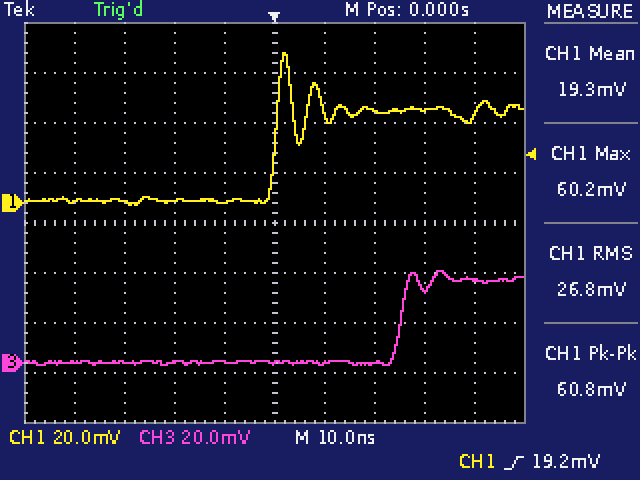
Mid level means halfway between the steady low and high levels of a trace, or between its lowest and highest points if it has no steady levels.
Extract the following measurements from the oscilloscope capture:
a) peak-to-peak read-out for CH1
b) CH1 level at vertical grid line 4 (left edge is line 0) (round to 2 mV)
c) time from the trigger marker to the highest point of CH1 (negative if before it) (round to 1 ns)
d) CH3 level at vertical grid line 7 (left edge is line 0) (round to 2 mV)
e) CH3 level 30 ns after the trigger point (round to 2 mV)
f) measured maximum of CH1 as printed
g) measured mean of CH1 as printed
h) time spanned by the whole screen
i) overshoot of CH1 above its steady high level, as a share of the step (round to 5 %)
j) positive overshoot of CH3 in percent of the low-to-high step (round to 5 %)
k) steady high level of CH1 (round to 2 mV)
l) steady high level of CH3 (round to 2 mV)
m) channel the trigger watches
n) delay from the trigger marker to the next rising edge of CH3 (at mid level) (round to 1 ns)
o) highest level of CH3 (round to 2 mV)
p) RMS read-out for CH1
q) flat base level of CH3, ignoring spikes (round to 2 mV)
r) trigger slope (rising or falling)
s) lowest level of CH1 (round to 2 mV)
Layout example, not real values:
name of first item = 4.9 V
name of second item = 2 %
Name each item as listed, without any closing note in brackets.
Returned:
peak-to-peak read-out for CH1 = 60.8 mV
CH1 level at vertical grid line 4 (left edge is line 0) = 0 mV
time from the trigger marker to the highest point of CH1 (negative if before it) = +2 ns
CH3 level at vertical grid line 7 (left edge is line 0) = 0 mV
CH3 level 30 ns after the trigger point = 30 mV
measured maximum of CH1 as printed = 60.2 mV
measured mean of CH1 as printed = 19.3 mV
time spanned by the whole screen = 100 ns
overshoot of CH1 above its steady high level, as a share of the step = 60 %
positive overshoot of CH3 in percent of the low-to-high step = 10 %
steady high level of CH1 = 38 mV
steady high level of CH3 = 34 mV
channel the trigger watches = CH1
delay from the trigger marker to the next rising edge of CH3 (at mid level) = 25 ns
highest level of CH3 = 36 mV
RMS read-out for CH1 = 26.8 mV
flat base level of CH3, ignoring spikes = 0 mV
trigger slope = rising
lowest level of CH1 = 0 mV
